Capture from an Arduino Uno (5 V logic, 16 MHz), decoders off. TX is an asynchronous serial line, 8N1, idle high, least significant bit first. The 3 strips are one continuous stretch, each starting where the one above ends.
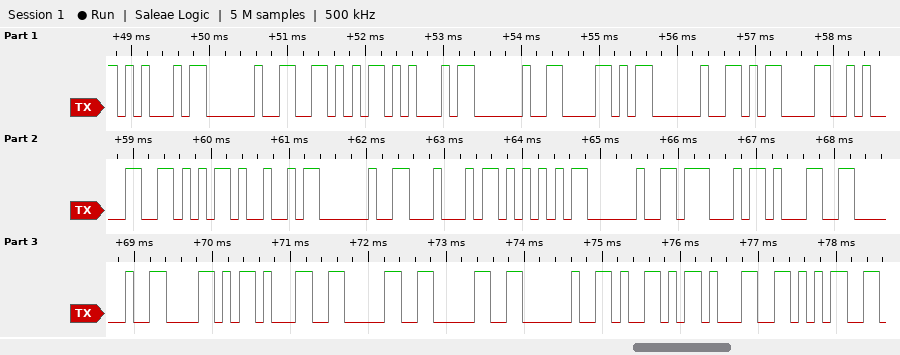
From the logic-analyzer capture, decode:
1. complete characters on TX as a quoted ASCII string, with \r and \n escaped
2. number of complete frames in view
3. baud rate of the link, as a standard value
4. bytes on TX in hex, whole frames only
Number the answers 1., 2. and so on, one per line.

1. "E VE X \r\nVI DU G1 X100 Y15"
2. 26
3. 9600 baud
4. 45 20 56 45 20 58 20 0D 0A 56 49 20 44 55 20 47 31 20 58 31 30 30 20 59 31 35
